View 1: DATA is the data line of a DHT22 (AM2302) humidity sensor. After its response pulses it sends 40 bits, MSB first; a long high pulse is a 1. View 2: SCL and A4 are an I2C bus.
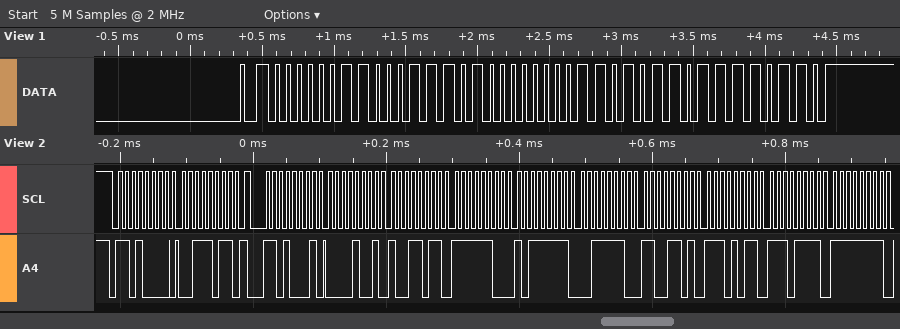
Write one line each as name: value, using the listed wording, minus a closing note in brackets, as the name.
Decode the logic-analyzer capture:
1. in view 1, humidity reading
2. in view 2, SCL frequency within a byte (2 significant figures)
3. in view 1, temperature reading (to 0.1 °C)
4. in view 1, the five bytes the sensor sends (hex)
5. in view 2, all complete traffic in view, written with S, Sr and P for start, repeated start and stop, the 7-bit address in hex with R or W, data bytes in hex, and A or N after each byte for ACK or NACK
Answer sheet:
in view 1, humidity reading: 79.7 %
in view 2, SCL frequency within a byte: 100 kHz
in view 1, temperature reading: 21.4 °C
in view 1, the five bytes the sensor sends: 03 1D 00 D6 F6
in view 2, all complete traffic in view, written with S, Sr and P for start, repeated start and stop, the 7-bit address in hex with R or W, data bytes in hex, and A or N after each byte for ACK or NACK: S 68W A 3B A Sr 68R A 09 A 9B A FC A BF A 3E A CD A EB A EF A FF A
